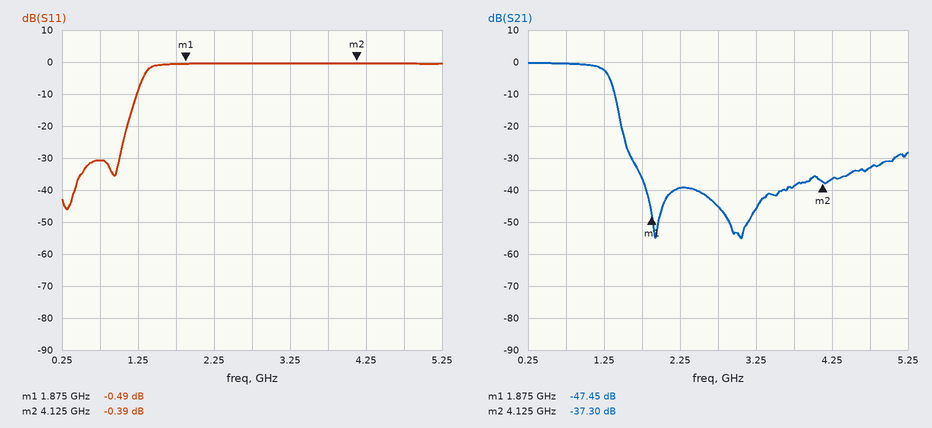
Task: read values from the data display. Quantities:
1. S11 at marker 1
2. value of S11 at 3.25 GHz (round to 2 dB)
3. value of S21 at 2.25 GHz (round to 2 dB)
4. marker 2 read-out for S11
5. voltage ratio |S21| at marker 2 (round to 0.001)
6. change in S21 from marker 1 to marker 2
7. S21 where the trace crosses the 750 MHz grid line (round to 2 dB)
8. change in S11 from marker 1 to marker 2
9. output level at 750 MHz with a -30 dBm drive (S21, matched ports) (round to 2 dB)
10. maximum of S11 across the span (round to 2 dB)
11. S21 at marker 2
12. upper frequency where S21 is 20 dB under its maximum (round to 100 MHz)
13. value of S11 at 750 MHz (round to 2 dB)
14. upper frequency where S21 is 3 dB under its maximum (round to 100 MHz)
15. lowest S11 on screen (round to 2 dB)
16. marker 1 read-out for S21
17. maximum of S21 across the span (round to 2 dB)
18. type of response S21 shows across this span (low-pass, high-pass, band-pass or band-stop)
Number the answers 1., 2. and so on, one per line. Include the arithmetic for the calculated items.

1. -0.49 dB
2. 0 dB
3. -40 dB
4. -0.39 dB
5. 10^(-37.3/20) ≈ 0.014
6. -37.3 − (-47.45) = 10.15 dB
7. 0 dB
8. -0.39 − (-0.49) = 0.10 dB
9. -30 dBm + (0 dB) = -30 dBm
10. 0 dB
11. -37.30 dB
12. 1.5 GHz
13. -30 dB
14. 1.3 GHz
15. -46 dB
16. -47.45 dB
17. 0 dB
18. low-pass
